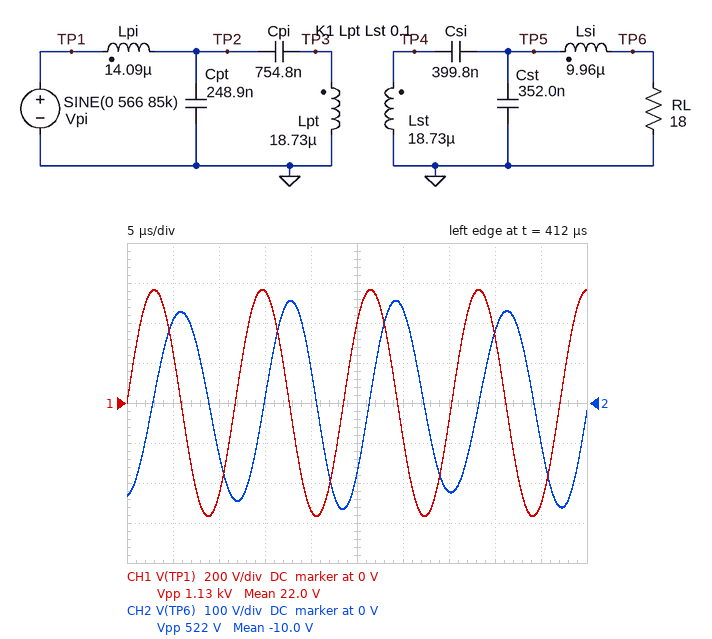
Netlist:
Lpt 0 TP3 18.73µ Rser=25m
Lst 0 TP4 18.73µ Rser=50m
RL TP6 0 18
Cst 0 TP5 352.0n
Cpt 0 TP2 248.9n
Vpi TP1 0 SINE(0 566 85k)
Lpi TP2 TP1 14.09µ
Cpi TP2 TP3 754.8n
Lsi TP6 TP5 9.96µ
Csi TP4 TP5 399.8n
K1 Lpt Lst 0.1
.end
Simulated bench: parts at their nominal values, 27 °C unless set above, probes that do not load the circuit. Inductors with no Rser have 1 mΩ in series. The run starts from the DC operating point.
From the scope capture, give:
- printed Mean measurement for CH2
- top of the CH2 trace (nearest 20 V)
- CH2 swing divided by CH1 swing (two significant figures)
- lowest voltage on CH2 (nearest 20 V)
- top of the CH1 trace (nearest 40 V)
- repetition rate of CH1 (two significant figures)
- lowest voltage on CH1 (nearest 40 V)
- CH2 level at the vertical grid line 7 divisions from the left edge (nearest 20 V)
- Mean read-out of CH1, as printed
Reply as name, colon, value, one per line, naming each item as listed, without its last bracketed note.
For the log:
printed Mean measurement for CH2: -10.0 V
top of the CH2 trace: 260 V
CH2 swing divided by CH1 swing: 0.46
lowest voltage on CH2: -260 V
top of the CH1 trace: 560 V
repetition rate of CH1: 85 kHz
lowest voltage on CH1: -560 V
CH2 level at the vertical grid line 7 divisions from the left edge: -220 V
Mean read-out of CH1, as printed: 22.0 V
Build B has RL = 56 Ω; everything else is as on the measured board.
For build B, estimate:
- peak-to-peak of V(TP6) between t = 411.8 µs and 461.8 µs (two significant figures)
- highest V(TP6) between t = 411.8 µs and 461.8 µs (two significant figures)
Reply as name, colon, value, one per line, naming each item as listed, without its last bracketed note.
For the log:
peak-to-peak of V(TP6) between t = 411.8 µs and 461.8 µs: 1.5 kV
highest V(TP6) between t = 411.8 µs and 461.8 µs: 730 V
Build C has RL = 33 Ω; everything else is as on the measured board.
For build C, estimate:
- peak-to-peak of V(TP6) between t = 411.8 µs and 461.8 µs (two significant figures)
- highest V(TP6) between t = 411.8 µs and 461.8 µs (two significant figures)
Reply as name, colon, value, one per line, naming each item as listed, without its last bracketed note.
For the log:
peak-to-peak of V(TP6) between t = 411.8 µs and 461.8 µs: 910 V
highest V(TP6) between t = 411.8 µs and 461.8 µs: 450 V
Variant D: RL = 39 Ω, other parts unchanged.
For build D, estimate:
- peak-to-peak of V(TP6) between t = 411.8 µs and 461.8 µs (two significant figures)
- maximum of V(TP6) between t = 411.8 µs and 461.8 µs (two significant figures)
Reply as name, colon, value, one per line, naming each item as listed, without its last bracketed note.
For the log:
peak-to-peak of V(TP6) between t = 411.8 µs and 461.8 µs: 1.1 kV
maximum of V(TP6) between t = 411.8 µs and 461.8 µs: 530 V
